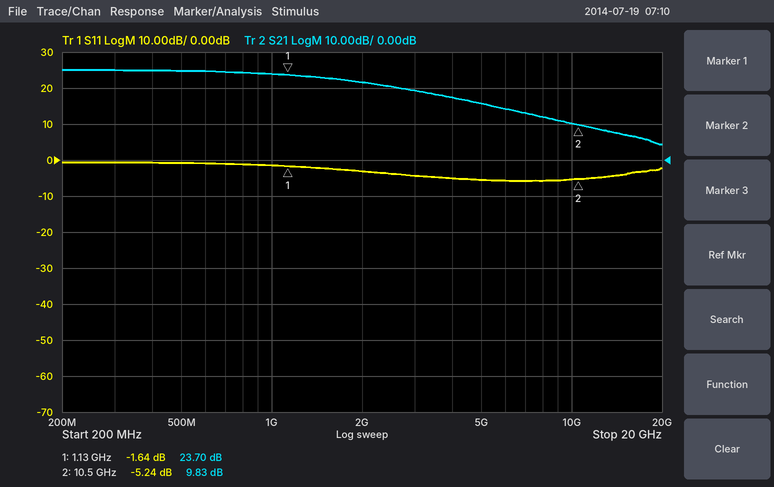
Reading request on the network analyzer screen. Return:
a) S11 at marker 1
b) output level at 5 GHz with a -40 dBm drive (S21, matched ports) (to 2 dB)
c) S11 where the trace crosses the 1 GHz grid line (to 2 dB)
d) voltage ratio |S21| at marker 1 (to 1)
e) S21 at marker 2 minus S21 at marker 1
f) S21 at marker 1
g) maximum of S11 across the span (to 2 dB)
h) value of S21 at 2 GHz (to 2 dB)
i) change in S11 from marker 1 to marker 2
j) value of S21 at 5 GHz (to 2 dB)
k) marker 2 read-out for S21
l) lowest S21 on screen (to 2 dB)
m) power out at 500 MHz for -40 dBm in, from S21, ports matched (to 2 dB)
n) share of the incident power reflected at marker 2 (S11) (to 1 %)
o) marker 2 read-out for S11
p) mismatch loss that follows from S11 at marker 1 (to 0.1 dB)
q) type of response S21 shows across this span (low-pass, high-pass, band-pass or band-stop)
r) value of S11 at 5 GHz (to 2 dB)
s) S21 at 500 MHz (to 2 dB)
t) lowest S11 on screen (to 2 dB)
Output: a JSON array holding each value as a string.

["-1.64 dB", "-24 dBm", "-2 dB", "15", "-13.87 dB", "23.70 dB", "0 dB", "22 dB", "-3.60 dB", "16 dB", "9.83 dB", "4 dB", "-16 dBm", "30 %", "-5.24 dB", "5.0 dB", "low-pass", "-6 dB", "24 dB", "-6 dB"]
